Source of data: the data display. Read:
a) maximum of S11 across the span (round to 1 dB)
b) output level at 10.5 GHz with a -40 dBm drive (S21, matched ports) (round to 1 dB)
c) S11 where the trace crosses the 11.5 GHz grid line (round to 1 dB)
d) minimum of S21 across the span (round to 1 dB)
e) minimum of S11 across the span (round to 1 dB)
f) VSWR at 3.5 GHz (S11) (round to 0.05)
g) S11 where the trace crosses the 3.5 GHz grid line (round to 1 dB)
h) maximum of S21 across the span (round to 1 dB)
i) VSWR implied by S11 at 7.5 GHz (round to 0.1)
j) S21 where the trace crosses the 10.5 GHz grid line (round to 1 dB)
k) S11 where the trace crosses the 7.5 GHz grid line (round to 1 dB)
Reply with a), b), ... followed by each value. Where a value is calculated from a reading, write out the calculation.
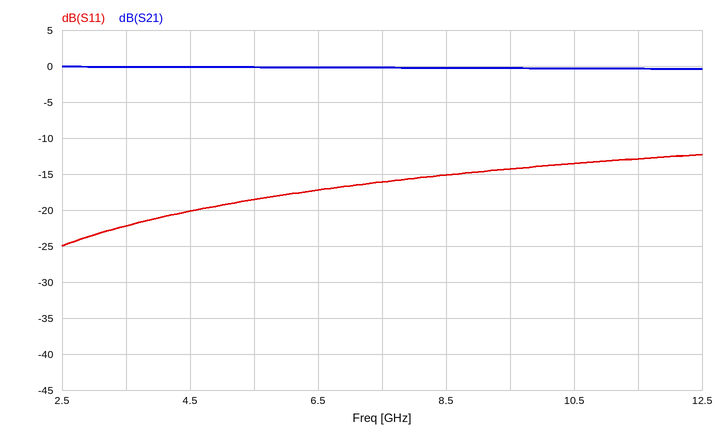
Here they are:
a) -12 dB
b) -40 dBm + (0 dB) = -40 dBm
c) -13 dB
d) 0 dB
e) -25 dB
f) |Γ| = 10^(-22/20) = 0.0794; VSWR = (1 + 0.0794)/(1 − 0.0794) ≈ 1.17, so 1.15 to the nearest 0.05
g) -22 dB
h) 0 dB
i) |Γ| = 10^(-16/20) = 0.1585; VSWR = (1 + 0.1585)/(1 − 0.1585) ≈ 1.4
j) 0 dB
k) -16 dB
